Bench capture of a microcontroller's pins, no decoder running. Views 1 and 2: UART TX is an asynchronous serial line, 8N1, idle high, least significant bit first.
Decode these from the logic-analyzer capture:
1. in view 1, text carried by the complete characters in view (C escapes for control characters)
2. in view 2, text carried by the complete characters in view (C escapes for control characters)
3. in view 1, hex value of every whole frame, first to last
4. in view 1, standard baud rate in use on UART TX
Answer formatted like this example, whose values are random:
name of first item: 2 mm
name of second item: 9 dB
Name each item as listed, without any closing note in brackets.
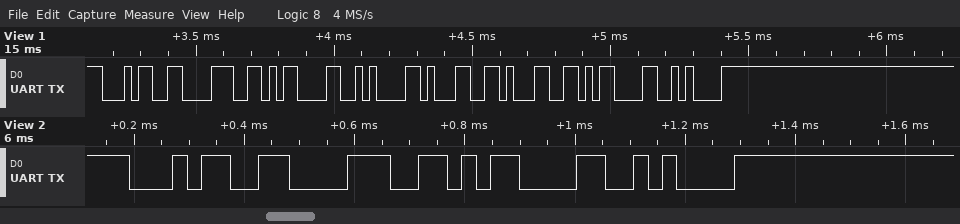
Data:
in view 1, text carried by the complete characters in view: "48\r\n11\r\n"
in view 2, text carried by the complete characters in view: "48\r\n"
in view 1, hex value of every whole frame, first to last: 34 38 0D 0A 31 31 0D 0A
in view 1, standard baud rate in use on UART TX: 38400 baud
